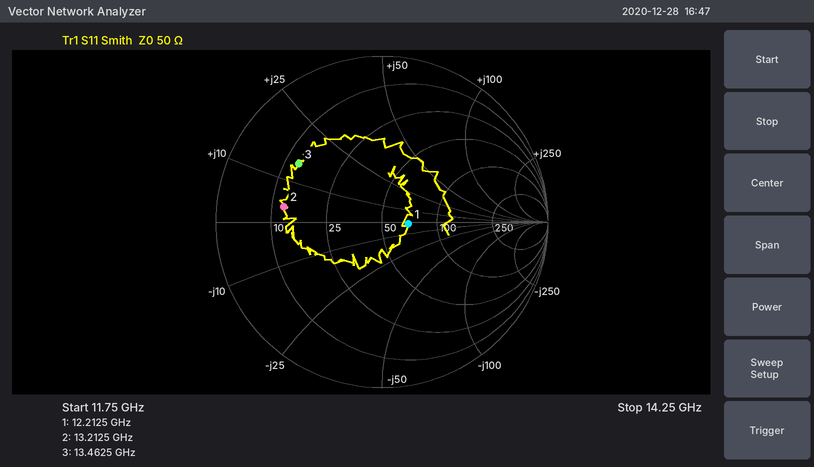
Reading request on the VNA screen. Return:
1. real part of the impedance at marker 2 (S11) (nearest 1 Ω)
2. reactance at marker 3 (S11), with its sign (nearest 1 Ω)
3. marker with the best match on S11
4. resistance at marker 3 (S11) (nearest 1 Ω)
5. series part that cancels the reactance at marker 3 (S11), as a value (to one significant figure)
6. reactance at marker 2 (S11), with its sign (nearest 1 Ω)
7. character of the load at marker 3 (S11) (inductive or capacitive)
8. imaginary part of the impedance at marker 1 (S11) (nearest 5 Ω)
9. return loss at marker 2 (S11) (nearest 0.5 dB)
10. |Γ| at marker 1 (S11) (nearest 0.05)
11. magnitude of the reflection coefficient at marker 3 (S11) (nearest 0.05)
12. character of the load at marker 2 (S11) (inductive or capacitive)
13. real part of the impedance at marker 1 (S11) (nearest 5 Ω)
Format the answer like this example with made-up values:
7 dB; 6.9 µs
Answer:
13 Ω; +15 Ω; marker 1; 13 Ω; 800 fF; +4 Ω; inductive; 0 Ω; 4.5 dB; 0.15; 0.60; inductive; 70 Ω
